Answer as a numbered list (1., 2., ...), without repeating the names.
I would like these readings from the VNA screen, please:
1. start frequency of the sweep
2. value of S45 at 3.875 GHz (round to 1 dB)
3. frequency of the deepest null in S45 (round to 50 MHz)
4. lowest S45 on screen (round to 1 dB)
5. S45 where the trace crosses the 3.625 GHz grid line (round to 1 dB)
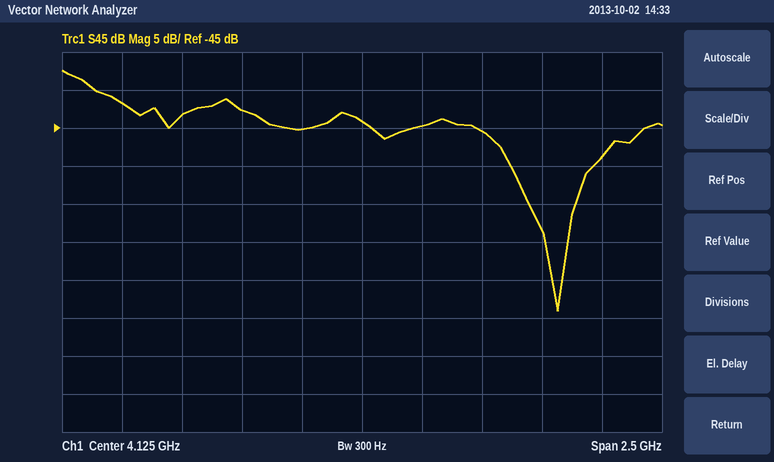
1. 2.875 GHz
2. -45 dB
3. 4.95 GHz
4. -69 dB
5. -43 dB
